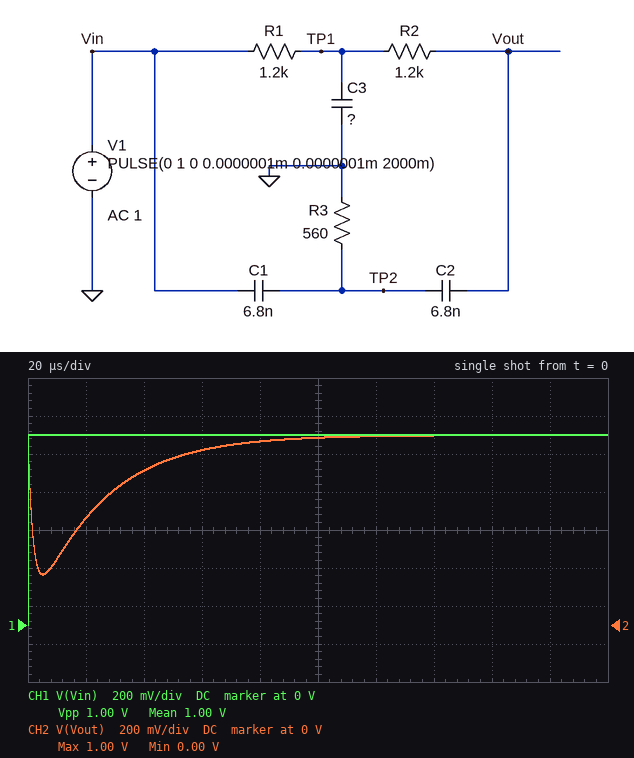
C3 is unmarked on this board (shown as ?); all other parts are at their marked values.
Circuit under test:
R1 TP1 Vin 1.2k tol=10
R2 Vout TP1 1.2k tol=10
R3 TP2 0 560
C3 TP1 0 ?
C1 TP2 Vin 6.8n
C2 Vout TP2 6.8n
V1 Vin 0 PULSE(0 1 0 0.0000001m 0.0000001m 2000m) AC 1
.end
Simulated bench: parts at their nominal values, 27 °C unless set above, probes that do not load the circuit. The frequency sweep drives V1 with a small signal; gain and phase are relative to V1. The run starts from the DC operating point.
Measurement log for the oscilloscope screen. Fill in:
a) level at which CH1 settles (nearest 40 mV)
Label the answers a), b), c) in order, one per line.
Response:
a) 1.00 V
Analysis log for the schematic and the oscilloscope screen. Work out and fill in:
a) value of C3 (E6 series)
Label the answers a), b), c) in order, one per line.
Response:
a) 4.7 nF
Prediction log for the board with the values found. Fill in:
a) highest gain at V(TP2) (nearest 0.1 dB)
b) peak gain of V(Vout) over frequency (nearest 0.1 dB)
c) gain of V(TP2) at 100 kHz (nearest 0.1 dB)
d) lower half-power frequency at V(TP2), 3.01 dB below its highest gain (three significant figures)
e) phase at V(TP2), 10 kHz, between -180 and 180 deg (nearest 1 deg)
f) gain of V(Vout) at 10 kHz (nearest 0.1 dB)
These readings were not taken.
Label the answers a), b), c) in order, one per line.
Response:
a) 0 dB
b) 0 dB
c) -2.0 dB
d) 71.1 kHz
e) 50 deg
f) -6.6 dB
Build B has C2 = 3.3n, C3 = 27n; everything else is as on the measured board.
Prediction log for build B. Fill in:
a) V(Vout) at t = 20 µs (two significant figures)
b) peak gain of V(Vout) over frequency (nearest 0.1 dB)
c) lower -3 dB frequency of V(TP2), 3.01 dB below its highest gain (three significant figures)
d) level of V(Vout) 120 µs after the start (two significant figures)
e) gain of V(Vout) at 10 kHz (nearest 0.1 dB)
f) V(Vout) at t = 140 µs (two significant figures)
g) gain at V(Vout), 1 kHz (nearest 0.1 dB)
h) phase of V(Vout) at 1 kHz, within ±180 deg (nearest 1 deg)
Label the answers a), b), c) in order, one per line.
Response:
a) 340 mV
b) 0 dB
c) 67.8 kHz
d) 960 mV
e) -9.7 dB
f) 970 mV
g) -0.2 dB
h) -14 deg
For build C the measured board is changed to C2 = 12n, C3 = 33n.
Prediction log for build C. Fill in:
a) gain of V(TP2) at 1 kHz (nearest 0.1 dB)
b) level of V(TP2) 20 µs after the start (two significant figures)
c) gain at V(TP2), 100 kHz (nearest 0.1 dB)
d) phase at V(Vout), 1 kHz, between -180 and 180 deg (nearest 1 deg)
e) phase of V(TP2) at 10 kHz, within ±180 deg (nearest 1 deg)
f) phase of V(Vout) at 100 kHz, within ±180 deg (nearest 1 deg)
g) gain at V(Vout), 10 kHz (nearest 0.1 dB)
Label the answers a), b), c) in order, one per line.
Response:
a) -24.2 dB
b) 92 mV
c) -1.6 dB
d) -24 deg
e) 46 deg
f) 37 deg
g) -19.6 dB
